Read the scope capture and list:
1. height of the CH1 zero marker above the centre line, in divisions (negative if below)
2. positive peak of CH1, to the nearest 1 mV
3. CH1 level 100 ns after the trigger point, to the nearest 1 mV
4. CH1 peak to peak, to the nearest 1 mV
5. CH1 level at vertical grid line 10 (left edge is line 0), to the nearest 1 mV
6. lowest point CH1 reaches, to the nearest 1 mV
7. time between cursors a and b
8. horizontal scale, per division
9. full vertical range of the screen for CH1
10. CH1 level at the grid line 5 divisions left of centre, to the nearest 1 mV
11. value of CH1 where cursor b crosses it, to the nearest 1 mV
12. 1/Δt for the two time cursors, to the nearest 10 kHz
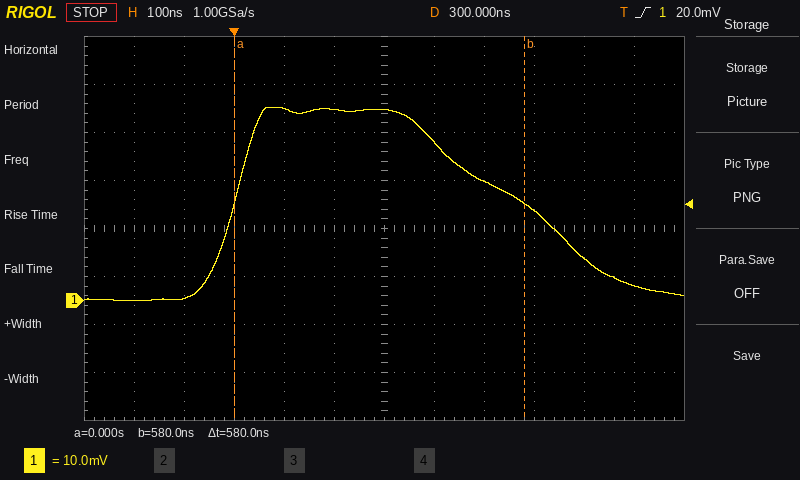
-1.5 div
40 mV
40 mV
40 mV
9 mV
0 mV
580 ns
100 ns
80 mV
0 mV
20 mV
1.72 MHz
